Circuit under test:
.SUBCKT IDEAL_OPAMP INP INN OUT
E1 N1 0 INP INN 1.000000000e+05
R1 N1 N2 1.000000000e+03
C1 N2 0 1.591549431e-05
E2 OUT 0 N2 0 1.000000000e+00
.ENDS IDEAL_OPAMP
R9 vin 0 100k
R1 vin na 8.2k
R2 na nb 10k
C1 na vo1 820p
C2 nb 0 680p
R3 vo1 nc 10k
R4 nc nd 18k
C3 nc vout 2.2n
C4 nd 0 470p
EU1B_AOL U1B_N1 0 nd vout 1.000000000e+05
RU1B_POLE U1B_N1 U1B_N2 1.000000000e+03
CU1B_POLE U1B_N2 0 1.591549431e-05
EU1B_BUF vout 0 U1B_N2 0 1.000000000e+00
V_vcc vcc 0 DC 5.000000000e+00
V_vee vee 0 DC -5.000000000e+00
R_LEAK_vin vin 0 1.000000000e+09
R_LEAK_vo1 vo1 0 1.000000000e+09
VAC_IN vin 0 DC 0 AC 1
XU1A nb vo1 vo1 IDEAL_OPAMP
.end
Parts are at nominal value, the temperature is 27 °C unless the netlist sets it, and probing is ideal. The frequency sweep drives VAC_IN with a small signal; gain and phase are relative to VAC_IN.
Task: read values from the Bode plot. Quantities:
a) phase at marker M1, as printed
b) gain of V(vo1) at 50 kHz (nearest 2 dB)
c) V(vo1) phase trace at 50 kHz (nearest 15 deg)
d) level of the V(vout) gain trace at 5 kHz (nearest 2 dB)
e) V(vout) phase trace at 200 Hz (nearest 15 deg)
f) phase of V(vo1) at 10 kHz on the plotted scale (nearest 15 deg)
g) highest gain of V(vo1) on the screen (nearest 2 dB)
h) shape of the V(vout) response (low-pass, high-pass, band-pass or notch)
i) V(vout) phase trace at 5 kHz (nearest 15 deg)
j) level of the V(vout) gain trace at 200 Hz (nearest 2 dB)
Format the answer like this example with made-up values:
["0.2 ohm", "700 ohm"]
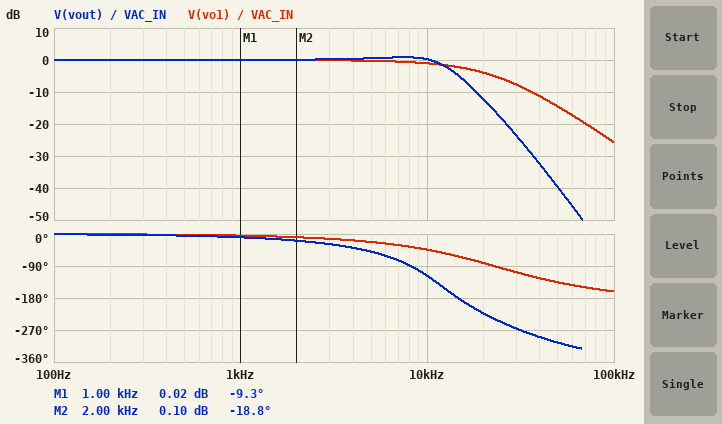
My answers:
["-9.3 deg", "-14 dB", "-135 deg", "0 dB", "0 deg", "-45 deg", "0 dB", "low-pass", "-45 deg", "0 dB"]
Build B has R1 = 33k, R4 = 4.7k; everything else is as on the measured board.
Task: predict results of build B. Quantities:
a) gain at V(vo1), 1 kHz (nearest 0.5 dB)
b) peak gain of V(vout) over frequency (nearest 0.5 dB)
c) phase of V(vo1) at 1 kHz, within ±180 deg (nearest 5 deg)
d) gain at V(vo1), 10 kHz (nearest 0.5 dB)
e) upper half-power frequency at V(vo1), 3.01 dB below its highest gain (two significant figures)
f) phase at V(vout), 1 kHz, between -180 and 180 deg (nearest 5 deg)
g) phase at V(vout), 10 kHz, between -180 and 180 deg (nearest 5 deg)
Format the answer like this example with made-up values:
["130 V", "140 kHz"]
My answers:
["0 dB", "0 dB", "-10 deg", "-5.5 dB", "6.8 kHz", "-15 deg", "-110 deg"]
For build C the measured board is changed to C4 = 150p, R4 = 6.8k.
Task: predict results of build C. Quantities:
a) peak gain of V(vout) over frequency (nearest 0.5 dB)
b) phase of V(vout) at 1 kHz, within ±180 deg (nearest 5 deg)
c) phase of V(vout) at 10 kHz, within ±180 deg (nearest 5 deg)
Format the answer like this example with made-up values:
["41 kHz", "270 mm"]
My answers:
["0 dB", "-5 deg", "-55 deg"]
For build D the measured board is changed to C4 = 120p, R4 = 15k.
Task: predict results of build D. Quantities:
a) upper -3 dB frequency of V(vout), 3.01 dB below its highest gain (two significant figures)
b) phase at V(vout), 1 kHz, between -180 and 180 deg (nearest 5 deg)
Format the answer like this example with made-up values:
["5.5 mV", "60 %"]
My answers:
["26 kHz", "-5 deg"]
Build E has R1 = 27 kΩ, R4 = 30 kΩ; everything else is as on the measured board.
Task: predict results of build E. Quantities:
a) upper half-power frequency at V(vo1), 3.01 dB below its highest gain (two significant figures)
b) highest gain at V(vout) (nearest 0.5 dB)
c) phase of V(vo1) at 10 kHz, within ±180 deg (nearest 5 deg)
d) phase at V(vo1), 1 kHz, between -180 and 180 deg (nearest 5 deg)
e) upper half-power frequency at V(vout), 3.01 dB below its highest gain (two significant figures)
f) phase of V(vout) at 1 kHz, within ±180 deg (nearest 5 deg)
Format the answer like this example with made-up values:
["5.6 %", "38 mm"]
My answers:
["8.1 kHz", "0 dB", "-75 deg", "-10 deg", "8.3 kHz", "-15 deg"]
